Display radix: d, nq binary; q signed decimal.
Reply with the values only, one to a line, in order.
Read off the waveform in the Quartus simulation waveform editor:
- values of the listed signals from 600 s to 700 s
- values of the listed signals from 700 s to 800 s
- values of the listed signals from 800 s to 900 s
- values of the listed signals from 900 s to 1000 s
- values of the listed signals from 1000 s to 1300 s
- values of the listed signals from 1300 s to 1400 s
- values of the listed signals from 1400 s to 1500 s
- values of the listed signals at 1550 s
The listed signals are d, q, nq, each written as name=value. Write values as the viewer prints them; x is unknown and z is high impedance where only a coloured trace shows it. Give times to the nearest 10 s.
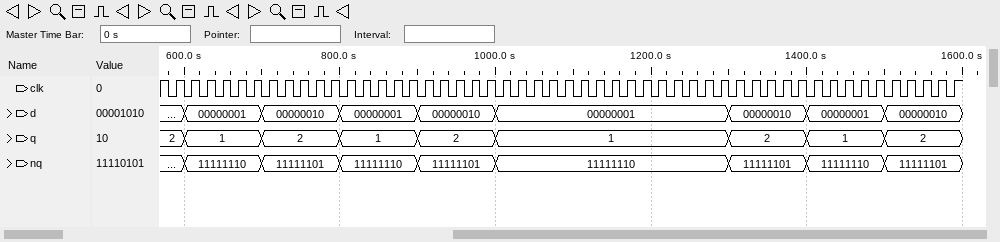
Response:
d=00000001, q=1, nq=11111110
d=00000010, q=2, nq=11111101
d=00000001, q=1, nq=11111110
d=00000010, q=2, nq=11111101
d=00000001, q=1, nq=11111110
d=00000010, q=2, nq=11111101
d=00000001, q=1, nq=11111110
d=00000010, q=2, nq=11111101
